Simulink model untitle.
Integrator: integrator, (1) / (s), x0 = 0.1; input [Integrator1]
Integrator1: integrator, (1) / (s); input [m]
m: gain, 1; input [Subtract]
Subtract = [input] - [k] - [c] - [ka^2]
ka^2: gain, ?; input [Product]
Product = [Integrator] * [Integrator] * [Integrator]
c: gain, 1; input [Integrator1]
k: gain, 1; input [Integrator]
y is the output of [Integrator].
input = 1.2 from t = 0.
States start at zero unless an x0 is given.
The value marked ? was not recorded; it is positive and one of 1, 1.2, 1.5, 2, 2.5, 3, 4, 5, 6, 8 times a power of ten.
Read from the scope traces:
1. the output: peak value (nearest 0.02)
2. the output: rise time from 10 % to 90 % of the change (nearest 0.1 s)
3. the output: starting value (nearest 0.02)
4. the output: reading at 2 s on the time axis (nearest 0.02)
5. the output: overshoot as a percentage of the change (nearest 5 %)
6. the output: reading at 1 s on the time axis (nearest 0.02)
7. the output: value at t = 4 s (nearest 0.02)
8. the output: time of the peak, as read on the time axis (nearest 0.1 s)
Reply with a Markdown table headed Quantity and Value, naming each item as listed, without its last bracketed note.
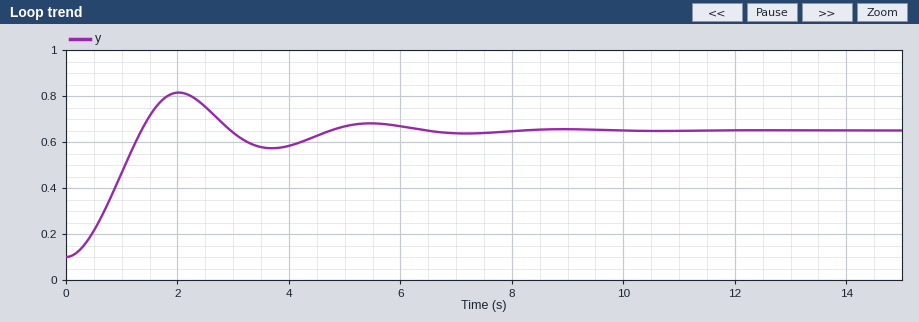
| Quantity | Value |
|---|---|
| the output: peak value | 0.82 |
| the output: rise time from 10 % to 90 % of the change | 0.9 s |
| the output: starting value | 0.10 |
| the output: reading at 2 s on the time axis | 0.82 |
| the output: overshoot as a percentage of the change | 30 % |
| the output: reading at 1 s on the time axis | 0.46 |
| the output: value at t = 4 s | 0.58 |
| the output: time of the peak, as read on the time axis | 2.0 s |
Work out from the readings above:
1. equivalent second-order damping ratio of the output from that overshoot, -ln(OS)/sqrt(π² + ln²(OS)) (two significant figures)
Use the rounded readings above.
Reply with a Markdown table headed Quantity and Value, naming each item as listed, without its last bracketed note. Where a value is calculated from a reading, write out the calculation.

| Quantity | Value |
|---|---|
| equivalent second-order damping ratio of the output from that overshoot, -ln(OS)/sqrt(π² + ln²(OS)) | ln(0.3) = -1.204; 1.204 / sqrt(9.870 + 1.450) = 0.36 |
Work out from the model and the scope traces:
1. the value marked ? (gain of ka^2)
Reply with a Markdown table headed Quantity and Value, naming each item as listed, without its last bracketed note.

| Quantity | Value |
|---|---|
| the value marked ? | 2 |
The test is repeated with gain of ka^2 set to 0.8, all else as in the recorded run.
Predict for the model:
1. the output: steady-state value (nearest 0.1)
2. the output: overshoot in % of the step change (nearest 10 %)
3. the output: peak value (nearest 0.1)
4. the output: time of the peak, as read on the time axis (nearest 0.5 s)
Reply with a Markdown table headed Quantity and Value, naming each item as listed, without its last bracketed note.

| Quantity | Value |
|---|---|
| the output: steady-state value | 0.8 |
| the output: overshoot in % of the step change | 30 % |
| the output: peak value | 1.0 |
| the output: time of the peak, as read on the time axis | 2.5 s |
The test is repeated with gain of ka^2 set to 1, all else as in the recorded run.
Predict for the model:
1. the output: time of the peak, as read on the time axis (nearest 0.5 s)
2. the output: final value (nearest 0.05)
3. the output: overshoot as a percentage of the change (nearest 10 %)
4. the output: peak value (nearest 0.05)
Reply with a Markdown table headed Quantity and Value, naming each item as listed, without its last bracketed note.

| Quantity | Value |
|---|---|
| the output: time of the peak, as read on the time axis | 2.5 s |
| the output: final value | 0.75 |
| the output: overshoot as a percentage of the change | 30 % |
| the output: peak value | 0.95 |
